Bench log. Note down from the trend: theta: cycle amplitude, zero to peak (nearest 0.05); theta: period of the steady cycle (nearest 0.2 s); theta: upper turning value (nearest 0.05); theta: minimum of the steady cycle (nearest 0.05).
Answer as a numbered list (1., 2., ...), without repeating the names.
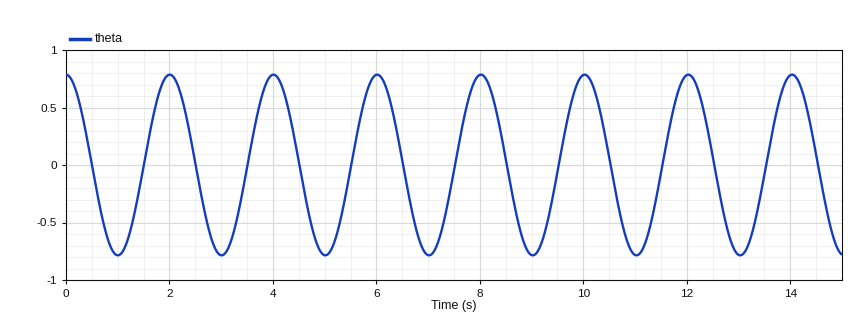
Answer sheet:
1. 0.80
2. 2.0 s
3. 0.80
4. -0.80
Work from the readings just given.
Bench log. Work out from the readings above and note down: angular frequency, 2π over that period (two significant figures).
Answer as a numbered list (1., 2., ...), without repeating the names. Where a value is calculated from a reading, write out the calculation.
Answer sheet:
1. 2π / 2 = 3.1 rad/s
